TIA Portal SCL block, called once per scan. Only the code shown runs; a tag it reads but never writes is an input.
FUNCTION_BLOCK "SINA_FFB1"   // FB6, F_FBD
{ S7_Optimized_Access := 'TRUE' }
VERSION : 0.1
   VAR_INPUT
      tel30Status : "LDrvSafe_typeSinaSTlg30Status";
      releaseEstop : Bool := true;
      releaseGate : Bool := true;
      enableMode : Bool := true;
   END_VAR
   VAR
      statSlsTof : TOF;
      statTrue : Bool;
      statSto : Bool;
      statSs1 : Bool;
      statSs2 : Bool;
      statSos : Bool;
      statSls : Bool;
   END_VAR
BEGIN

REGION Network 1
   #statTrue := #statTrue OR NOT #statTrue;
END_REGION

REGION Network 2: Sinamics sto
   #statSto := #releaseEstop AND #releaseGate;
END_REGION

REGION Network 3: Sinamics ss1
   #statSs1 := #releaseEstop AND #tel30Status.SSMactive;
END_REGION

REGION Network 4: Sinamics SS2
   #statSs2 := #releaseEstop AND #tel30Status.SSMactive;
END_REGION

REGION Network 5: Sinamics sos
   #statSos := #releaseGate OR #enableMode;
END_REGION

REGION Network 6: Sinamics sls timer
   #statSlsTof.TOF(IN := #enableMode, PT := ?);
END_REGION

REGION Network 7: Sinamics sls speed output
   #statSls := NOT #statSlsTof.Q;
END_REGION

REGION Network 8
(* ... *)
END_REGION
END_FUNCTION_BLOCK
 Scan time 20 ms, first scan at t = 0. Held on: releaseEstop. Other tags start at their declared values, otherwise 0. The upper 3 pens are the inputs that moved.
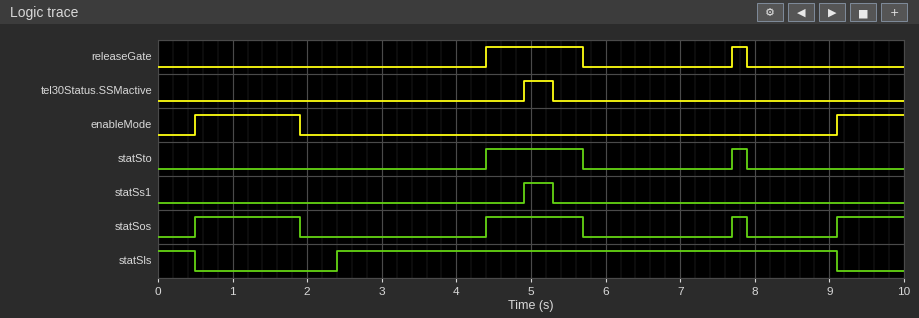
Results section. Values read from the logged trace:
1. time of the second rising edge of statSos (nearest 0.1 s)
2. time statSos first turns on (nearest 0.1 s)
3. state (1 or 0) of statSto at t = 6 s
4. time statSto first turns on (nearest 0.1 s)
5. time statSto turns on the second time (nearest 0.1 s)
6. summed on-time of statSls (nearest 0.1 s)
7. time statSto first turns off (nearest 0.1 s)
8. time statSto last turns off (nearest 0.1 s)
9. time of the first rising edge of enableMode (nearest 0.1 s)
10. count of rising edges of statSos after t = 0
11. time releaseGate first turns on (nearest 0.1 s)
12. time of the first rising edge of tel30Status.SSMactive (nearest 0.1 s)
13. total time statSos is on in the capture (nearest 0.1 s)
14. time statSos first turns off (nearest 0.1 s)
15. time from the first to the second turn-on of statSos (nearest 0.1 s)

4.4 s
0.5 s
0
4.4 s
7.7 s
7.2 s
5.7 s
7.9 s
0.5 s
4
4.4 s
4.9 s
3.8 s
1.9 s
3.9 s
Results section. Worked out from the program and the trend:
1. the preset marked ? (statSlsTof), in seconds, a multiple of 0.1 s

0.5 s
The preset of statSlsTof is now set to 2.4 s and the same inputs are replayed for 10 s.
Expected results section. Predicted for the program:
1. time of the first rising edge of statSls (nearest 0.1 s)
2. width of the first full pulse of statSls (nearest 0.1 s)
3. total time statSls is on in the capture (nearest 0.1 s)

4.3 s
4.8 s
5.3 s
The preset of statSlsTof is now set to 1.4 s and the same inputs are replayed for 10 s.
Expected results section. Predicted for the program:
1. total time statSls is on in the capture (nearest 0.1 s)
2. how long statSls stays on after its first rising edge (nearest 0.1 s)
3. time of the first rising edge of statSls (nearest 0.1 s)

6.3 s
5.8 s
3.3 s
